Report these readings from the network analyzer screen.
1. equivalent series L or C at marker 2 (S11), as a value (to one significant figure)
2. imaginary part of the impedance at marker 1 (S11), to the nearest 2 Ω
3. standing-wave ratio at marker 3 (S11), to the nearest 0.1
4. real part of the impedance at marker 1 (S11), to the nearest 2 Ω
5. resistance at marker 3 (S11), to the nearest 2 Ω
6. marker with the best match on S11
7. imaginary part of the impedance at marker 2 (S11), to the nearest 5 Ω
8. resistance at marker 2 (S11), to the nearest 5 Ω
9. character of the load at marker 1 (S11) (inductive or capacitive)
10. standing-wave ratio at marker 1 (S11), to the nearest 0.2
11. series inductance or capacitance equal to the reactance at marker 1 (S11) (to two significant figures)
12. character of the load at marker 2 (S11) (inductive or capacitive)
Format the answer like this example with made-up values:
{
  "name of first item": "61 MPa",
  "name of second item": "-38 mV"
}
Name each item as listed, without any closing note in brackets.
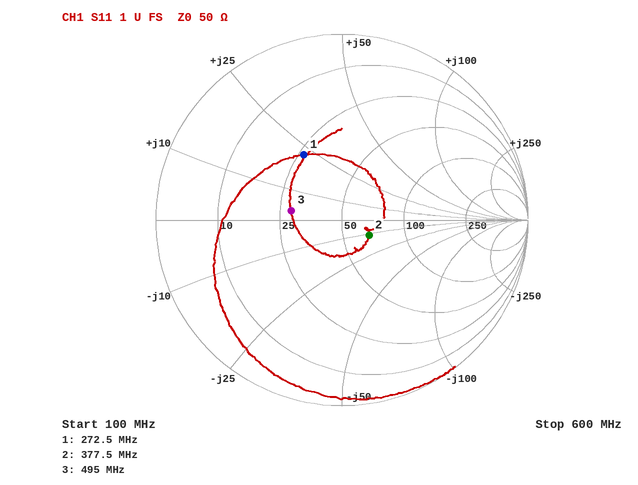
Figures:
{
  "equivalent series L or C at marker 2 (S11), as a value": "40 pF",
  "imaginary part of the impedance at marker 1 (S11), to the nearest 2 Ω": "+22 Ω",
  "standing-wave ratio at marker 3 (S11), to the nearest 0.1": "1.8",
  "real part of the impedance at marker 1 (S11), to the nearest 2 Ω": "26 Ω",
  "resistance at marker 3 (S11), to the nearest 2 Ω": "28 Ω",
  "marker with the best match on S11": "marker 2",
  "imaginary part of the impedance at marker 2 (S11), to the nearest 5 Ω": "-10 Ω",
  "resistance at marker 2 (S11), to the nearest 5 Ω": "65 Ω",
  "character of the load at marker 1 (S11)": "inductive",
  "standing-wave ratio at marker 1 (S11), to the nearest 0.2": "2.4",
  "series inductance or capacitance equal to the reactance at marker 1 (S11)": "13 nH",
  "character of the load at marker 2 (S11)": "capacitive"
}
